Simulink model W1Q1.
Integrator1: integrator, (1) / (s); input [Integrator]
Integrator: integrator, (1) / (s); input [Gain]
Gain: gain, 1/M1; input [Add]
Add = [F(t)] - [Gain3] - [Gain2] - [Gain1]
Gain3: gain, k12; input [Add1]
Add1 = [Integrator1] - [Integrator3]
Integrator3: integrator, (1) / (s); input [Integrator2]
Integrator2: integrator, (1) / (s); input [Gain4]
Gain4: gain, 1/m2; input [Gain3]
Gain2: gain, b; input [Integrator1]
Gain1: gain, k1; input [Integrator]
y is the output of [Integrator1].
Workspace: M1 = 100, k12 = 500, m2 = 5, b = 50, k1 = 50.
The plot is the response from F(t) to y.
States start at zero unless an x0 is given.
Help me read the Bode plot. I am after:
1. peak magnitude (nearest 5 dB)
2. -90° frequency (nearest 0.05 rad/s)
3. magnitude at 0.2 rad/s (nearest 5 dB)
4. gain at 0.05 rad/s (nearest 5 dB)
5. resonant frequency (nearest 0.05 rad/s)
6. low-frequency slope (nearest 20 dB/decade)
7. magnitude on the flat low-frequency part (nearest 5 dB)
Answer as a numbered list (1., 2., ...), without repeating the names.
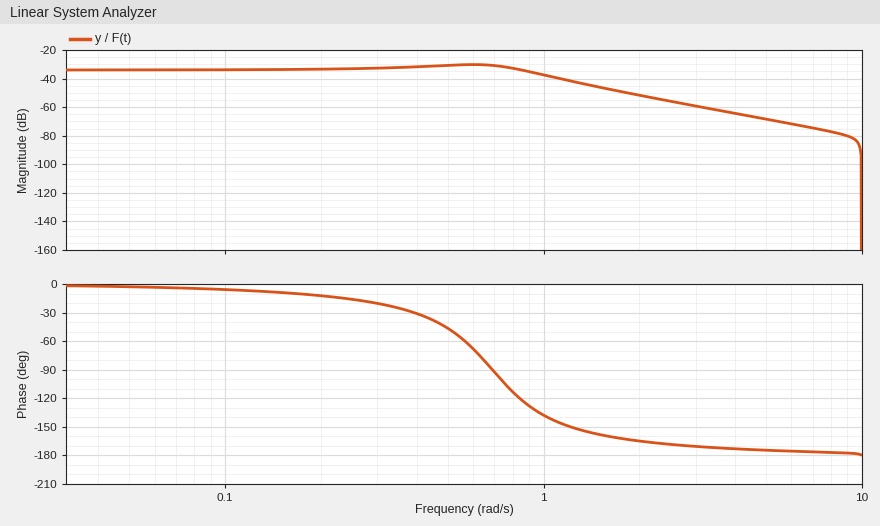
1. -30 dB
2. 0.70 rad/s
3. -35 dB
4. -35 dB
5. 0.60 rad/s
6. 0 dB/decade
7. -35 dB
